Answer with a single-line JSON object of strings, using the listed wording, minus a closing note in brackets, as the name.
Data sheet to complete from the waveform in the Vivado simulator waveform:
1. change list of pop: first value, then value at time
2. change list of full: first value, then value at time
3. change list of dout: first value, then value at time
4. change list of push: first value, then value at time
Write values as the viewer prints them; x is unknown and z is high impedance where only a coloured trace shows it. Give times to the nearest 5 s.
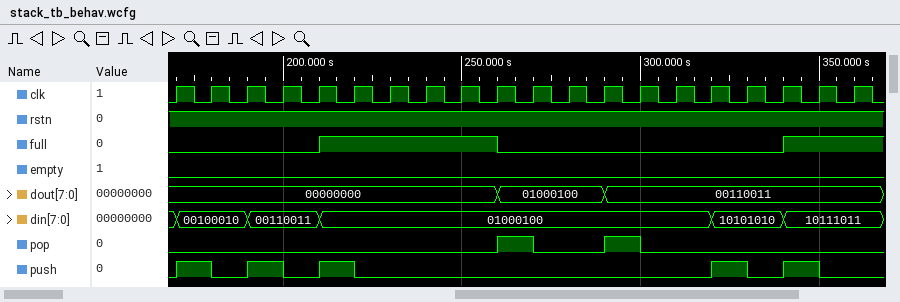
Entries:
{"change list of pop: first value, then value at time": "0, 1 at 260 s, 0 at 270 s, 1 at 290 s, 0 at 300 s", "change list of full: first value, then value at time": "0, 1 at 210 s, 0 at 260 s, 1 at 340 s", "change list of dout: first value, then value at time": "00000000, 01000100 at 260 s, 00110011 at 290 s", "change list of push: first value, then value at time": "0, 1 at 170 s, 0 at 180 s, 1 at 190 s, 0 at 200 s, 1 at 210 s, 0 at 220 s, 1 at 320 s, 0 at 330 s, 1 at 340 s, 0 at 350 s"}
